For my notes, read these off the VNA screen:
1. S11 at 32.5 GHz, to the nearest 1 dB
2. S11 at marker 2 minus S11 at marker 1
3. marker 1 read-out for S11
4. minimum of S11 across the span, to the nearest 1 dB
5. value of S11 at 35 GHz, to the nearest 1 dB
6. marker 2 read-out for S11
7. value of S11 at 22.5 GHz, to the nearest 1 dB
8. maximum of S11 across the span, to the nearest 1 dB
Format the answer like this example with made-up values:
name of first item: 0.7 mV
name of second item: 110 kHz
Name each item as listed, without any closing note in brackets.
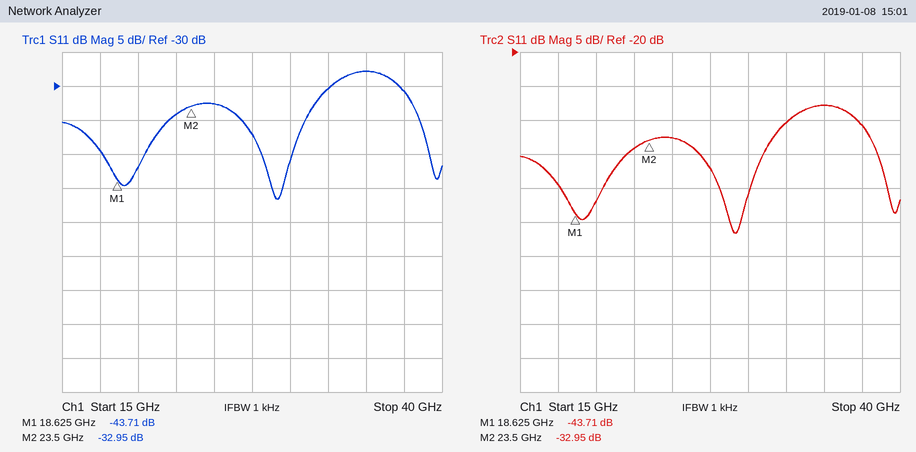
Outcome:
S11 at 32.5 GHz, to the nearest 1 dB: -30 dB
S11 at marker 2 minus S11 at marker 1: 10.76 dB
marker 1 read-out for S11: -43.71 dB
minimum of S11 across the span, to the nearest 1 dB: -47 dB
value of S11 at 35 GHz, to the nearest 1 dB: -28 dB
marker 2 read-out for S11: -32.95 dB
value of S11 at 22.5 GHz, to the nearest 1 dB: -34 dB
maximum of S11 across the span, to the nearest 1 dB: -28 dB
